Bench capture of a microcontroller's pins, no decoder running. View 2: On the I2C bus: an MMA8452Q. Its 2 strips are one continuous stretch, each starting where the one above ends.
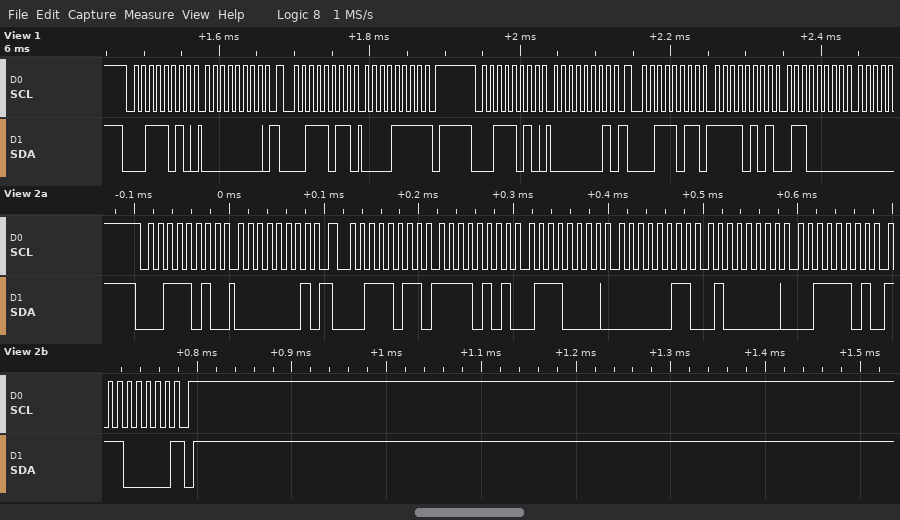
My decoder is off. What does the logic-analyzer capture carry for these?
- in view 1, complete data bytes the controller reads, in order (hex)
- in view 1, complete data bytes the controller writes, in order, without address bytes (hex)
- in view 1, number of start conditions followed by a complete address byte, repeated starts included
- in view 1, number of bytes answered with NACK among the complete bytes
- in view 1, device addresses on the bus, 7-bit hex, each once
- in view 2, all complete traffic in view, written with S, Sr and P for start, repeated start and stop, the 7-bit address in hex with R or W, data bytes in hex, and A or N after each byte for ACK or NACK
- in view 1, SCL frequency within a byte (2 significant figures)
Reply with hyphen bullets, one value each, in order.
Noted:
- 0F F5 60
- 00 01
- 4
- 1
- 0x1D
- S 1DW A 01 A Sr 1DR A F5 A 70 A 03 A 40 A 3D A E0 N P
- 100 kHz
